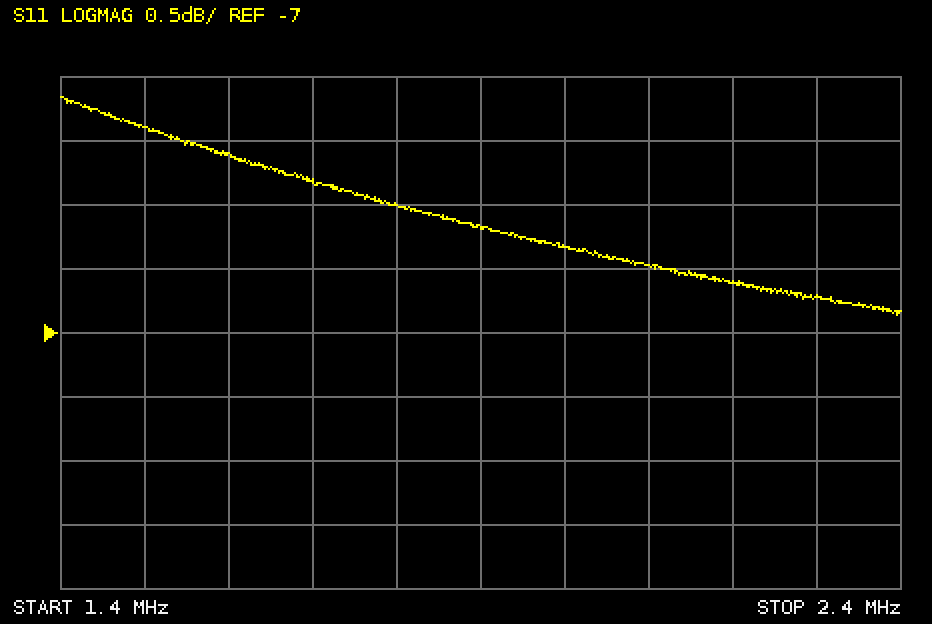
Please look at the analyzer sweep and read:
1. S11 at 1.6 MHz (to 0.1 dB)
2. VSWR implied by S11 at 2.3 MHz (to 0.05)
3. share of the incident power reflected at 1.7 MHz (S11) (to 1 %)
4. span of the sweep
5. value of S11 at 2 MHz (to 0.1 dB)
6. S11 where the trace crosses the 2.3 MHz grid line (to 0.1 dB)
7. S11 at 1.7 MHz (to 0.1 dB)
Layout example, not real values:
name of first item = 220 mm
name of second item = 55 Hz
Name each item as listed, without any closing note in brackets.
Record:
S11 at 1.6 MHz = -5.6 dB
VSWR implied by S11 at 2.3 MHz = 2.70
share of the incident power reflected at 1.7 MHz (S11) = 26 %
span of the sweep = 1 MHz
value of S11 at 2 MHz = -6.3 dB
S11 where the trace crosses the 2.3 MHz grid line = -6.7 dB
S11 at 1.7 MHz = -5.8 dB
